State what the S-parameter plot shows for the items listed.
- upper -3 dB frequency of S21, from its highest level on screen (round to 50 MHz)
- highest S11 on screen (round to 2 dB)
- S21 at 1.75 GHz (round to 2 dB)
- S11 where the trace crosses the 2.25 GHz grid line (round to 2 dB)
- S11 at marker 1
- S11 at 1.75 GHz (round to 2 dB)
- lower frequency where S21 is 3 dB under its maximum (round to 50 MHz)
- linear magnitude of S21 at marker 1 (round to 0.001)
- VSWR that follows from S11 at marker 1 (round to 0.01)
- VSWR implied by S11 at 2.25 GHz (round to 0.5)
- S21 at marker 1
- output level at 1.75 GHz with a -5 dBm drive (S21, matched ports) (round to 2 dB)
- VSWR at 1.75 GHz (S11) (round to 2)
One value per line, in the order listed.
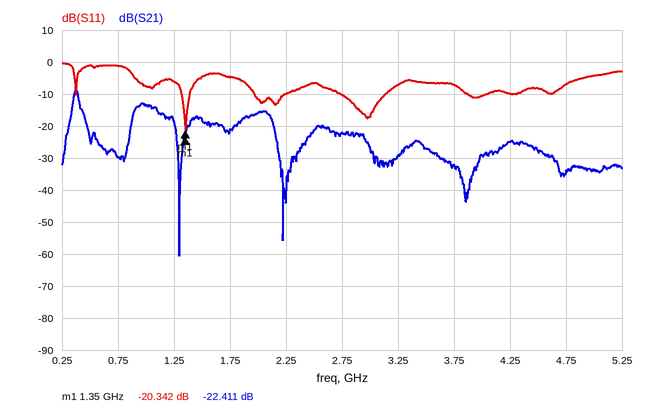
400 MHz
0 dB
-22 dB
-10 dB
-20.342 dB
-4 dB
350 MHz
0.076
1.21
2.0
-22.411 dB
-26 dBm
4
